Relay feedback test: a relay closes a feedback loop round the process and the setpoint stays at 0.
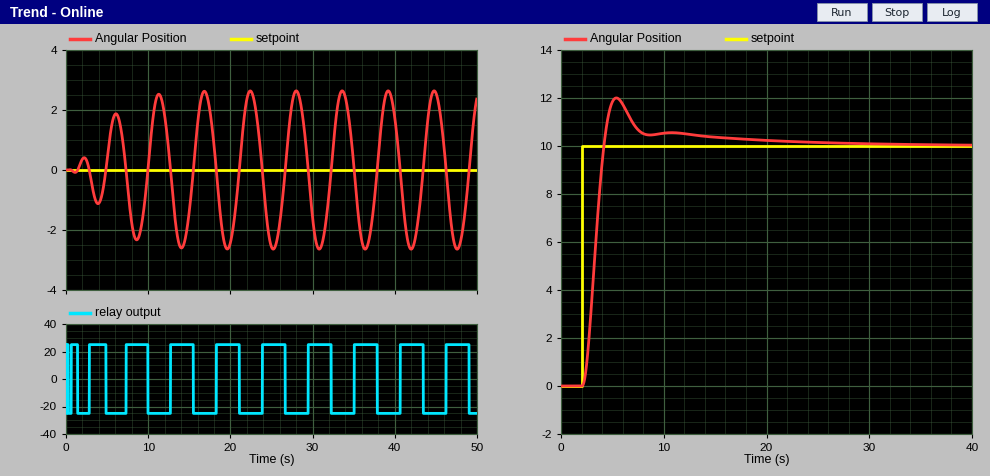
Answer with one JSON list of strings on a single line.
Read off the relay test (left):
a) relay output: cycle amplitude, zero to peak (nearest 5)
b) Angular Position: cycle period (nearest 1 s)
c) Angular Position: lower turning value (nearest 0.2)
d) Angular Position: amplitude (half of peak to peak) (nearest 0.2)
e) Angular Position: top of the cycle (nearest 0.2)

["25", "6 s", "-2.6", "2.6", "2.6"]
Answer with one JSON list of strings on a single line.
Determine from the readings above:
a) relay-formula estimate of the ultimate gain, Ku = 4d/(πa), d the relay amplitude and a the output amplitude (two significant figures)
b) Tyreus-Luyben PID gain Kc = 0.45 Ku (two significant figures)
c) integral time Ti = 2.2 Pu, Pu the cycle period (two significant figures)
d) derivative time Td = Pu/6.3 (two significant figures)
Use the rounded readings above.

["12", "5.4", "13 s", "0.95 s"]
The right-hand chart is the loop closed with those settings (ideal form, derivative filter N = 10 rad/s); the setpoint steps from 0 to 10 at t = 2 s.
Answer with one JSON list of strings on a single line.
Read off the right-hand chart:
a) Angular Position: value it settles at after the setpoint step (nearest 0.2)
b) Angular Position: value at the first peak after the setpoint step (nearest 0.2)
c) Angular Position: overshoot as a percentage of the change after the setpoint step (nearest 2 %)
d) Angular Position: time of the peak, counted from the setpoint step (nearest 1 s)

["10.0", "12.0", "20 %", "3 s"]
